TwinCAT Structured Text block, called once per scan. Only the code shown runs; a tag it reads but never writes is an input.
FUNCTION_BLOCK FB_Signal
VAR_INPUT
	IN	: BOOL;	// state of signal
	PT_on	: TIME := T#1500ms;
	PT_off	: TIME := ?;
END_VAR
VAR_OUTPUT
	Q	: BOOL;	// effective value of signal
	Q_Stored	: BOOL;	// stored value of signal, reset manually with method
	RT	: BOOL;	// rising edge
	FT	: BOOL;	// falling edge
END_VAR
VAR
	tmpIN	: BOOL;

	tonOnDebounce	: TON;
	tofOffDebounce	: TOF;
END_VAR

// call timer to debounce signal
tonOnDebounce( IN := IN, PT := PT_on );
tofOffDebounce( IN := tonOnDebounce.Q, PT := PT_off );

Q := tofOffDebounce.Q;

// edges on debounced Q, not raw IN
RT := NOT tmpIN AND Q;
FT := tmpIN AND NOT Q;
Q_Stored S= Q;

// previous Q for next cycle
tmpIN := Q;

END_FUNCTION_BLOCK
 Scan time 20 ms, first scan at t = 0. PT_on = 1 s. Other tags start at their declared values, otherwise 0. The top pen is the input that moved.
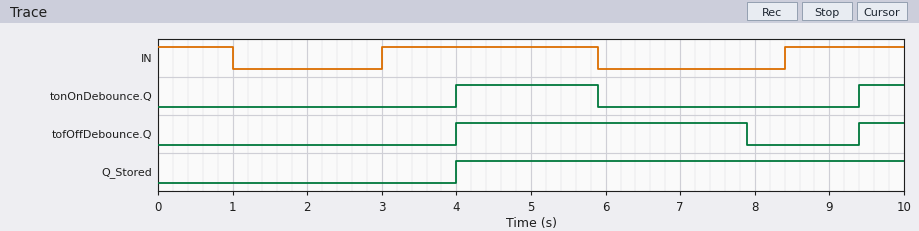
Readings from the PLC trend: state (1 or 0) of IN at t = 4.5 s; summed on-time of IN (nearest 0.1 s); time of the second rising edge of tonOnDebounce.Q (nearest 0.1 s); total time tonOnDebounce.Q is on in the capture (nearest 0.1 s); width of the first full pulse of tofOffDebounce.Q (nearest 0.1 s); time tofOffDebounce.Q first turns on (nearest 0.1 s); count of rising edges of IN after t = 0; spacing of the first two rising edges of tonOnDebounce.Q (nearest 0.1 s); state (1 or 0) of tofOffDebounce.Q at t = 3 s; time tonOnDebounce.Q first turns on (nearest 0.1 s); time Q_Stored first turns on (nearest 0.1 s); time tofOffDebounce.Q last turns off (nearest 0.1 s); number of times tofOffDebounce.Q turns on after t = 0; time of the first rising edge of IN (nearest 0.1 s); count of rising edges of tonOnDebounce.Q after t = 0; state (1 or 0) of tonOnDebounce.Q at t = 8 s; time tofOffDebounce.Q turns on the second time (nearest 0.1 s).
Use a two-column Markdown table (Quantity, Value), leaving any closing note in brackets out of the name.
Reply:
| Quantity | Value |
|---|---|
| state (1 or 0) of IN at t = 4.5 s | 1 |
| summed on-time of IN | 5.5 s |
| time of the second rising edge of tonOnDebounce.Q | 9.4 s |
| total time tonOnDebounce.Q is on in the capture | 2.5 s |
| width of the first full pulse of tofOffDebounce.Q | 3.9 s |
| time tofOffDebounce.Q first turns on | 4.0 s |
| count of rising edges of IN after t = 0 | 2 |
| spacing of the first two rising edges of tonOnDebounce.Q | 5.4 s |
| state (1 or 0) of tofOffDebounce.Q at t = 3 s | 0 |
| time tonOnDebounce.Q first turns on | 4.0 s |
| time Q_Stored first turns on | 4.0 s |
| time tofOffDebounce.Q last turns off | 7.9 s |
| number of times tofOffDebounce.Q turns on after t = 0 | 2 |
| time of the first rising edge of IN | 3.0 s |
| count of rising edges of tonOnDebounce.Q after t = 0 | 2 |
| state (1 or 0) of tonOnDebounce.Q at t = 8 s | 0 |
| time tofOffDebounce.Q turns on the second time | 9.4 s |
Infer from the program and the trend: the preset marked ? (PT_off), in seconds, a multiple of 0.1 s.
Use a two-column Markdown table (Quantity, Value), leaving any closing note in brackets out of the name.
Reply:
| Quantity | Value |
|---|---|
| the preset marked ? (PT_off), in seconds, a multiple of 0.1 s | 2.0 s |
